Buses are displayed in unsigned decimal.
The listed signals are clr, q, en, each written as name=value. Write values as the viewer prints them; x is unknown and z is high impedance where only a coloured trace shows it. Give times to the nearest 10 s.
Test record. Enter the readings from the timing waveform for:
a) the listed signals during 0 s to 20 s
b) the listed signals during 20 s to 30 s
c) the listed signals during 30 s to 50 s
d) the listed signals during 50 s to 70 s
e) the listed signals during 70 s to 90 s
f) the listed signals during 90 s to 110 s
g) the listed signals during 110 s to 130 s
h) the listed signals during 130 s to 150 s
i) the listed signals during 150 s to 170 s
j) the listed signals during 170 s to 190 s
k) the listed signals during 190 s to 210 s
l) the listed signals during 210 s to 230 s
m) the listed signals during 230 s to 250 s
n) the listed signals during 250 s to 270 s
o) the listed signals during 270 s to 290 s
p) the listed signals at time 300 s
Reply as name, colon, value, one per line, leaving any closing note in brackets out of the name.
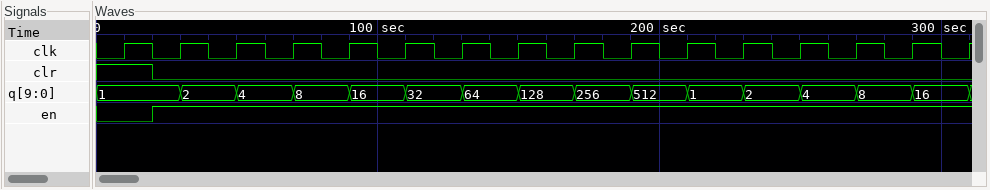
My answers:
the listed signals during 0 s to 20 s: clr=1, q=1, en=0
the listed signals during 20 s to 30 s: clr=0, q=1, en=1
the listed signals during 30 s to 50 s: clr=0, q=2, en=1
the listed signals during 50 s to 70 s: clr=0, q=4, en=1
the listed signals during 70 s to 90 s: clr=0, q=8, en=1
the listed signals during 90 s to 110 s: clr=0, q=16, en=1
the listed signals during 110 s to 130 s: clr=0, q=32, en=1
the listed signals during 130 s to 150 s: clr=0, q=64, en=1
the listed signals during 150 s to 170 s: clr=0, q=128, en=1
the listed signals during 170 s to 190 s: clr=0, q=256, en=1
the listed signals during 190 s to 210 s: clr=0, q=512, en=1
the listed signals during 210 s to 230 s: clr=0, q=1, en=1
the listed signals during 230 s to 250 s: clr=0, q=2, en=1
the listed signals during 250 s to 270 s: clr=0, q=4, en=1
the listed signals during 270 s to 290 s: clr=0, q=8, en=1
the listed signals at time 300 s: clr=0, q=16, en=1
